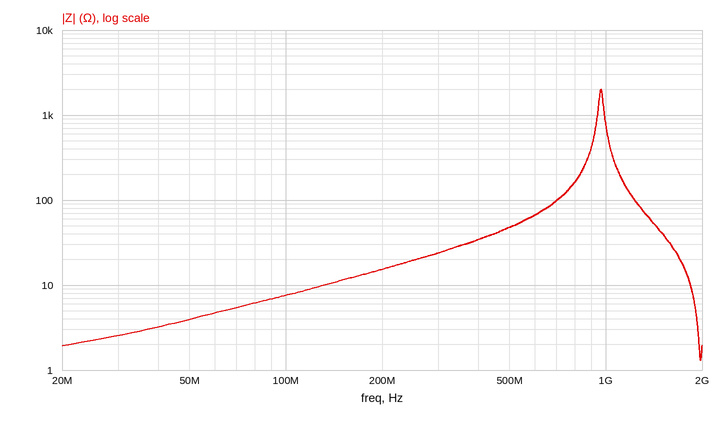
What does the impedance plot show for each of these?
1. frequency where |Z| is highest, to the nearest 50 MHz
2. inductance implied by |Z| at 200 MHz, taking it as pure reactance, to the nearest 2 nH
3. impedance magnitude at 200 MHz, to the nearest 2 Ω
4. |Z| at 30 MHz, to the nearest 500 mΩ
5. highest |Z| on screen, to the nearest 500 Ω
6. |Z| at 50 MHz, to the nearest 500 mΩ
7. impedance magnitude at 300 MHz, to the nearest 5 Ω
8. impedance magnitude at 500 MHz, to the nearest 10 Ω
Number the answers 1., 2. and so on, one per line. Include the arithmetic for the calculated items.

1. 950 MHz
2. L = 16 Ω/(2π × 200 MHz) ≈ 12.7 nH, so 12 nH to the nearest 2 nH
3. 16 Ω
4. 2.5 Ω
5. 2.0 kΩ
6. 4.0 Ω
7. 25 Ω
8. 50 Ω
